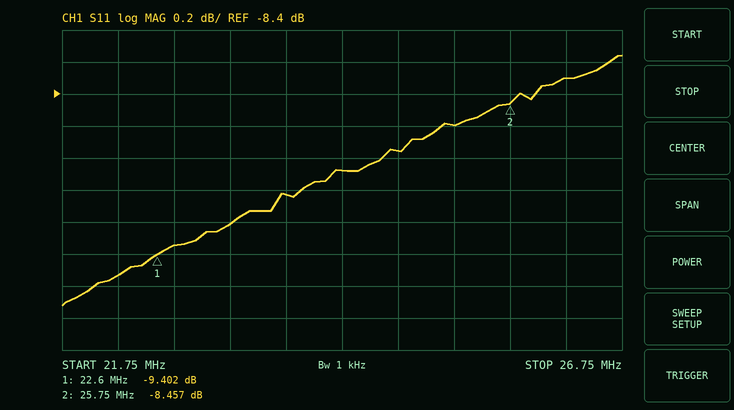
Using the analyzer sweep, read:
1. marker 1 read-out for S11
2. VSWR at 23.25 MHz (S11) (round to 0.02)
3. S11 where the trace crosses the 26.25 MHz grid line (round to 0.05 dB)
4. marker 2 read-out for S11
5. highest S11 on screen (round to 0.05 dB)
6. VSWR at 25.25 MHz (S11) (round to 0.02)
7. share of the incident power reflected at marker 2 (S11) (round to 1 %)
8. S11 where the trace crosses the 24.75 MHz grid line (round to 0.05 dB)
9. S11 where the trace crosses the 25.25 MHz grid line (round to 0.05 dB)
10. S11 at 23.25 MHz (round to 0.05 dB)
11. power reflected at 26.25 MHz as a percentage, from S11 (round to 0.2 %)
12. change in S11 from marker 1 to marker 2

-9.402 dB
2.06
-8.30 dB
-8.457 dB
-8.15 dB
2.18
14 %
-8.75 dB
-8.60 dB
-9.20 dB
14.8 %
0.945 dB
